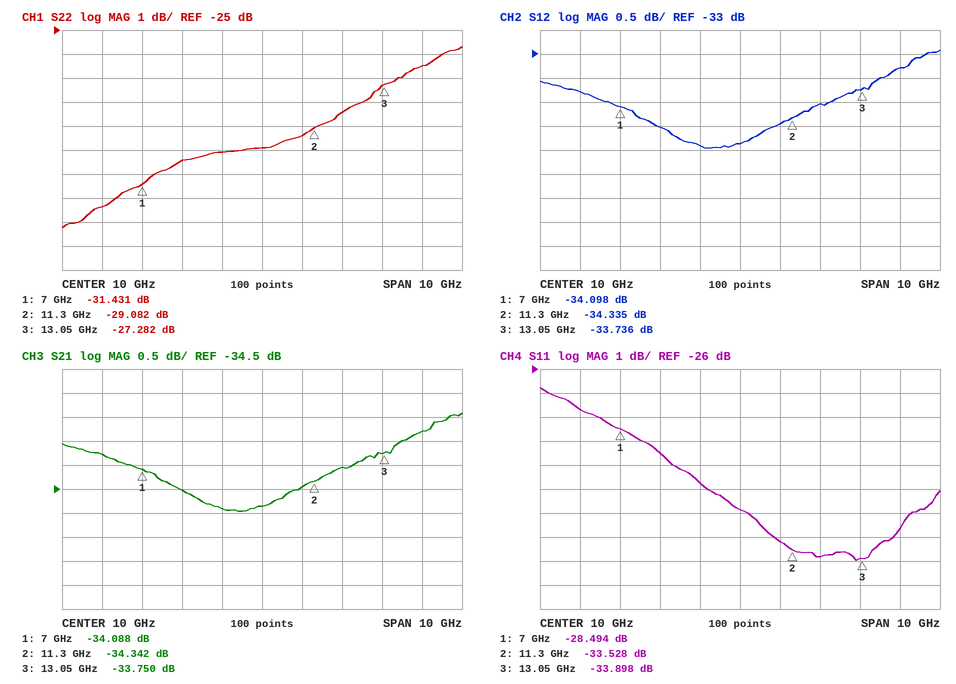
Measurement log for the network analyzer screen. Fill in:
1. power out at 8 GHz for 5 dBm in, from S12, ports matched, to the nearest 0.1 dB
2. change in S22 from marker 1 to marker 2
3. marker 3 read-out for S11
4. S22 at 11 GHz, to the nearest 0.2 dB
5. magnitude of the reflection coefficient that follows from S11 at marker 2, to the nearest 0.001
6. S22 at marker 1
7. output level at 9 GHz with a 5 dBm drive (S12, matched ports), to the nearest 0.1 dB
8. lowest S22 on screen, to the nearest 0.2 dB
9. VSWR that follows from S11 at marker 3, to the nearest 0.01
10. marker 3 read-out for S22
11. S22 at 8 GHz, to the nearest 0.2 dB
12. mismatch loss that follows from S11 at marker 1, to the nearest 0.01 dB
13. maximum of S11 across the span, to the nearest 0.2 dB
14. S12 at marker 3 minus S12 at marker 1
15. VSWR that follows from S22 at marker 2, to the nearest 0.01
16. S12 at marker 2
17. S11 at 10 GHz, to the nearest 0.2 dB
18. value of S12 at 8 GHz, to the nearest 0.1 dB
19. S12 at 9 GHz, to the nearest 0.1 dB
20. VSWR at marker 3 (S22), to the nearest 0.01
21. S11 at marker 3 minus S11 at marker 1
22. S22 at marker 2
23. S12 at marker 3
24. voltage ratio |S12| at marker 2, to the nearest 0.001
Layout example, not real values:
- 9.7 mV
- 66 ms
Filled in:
- -29.5 dBm
- 2.349 dB
- -33.898 dB
- -29.4 dB
- 0.021
- -31.431 dB
- -29.9 dBm
- -33.2 dB
- 1.04
- -27.282 dB
- -30.4 dB
- 0.01 dB
- -26.8 dB
- 0.362 dB
- 1.07
- -34.335 dB
- -31.8 dB
- -34.5 dB
- -34.9 dB
- 1.09
- -5.404 dB
- -29.082 dB
- -33.736 dB
- 0.019
